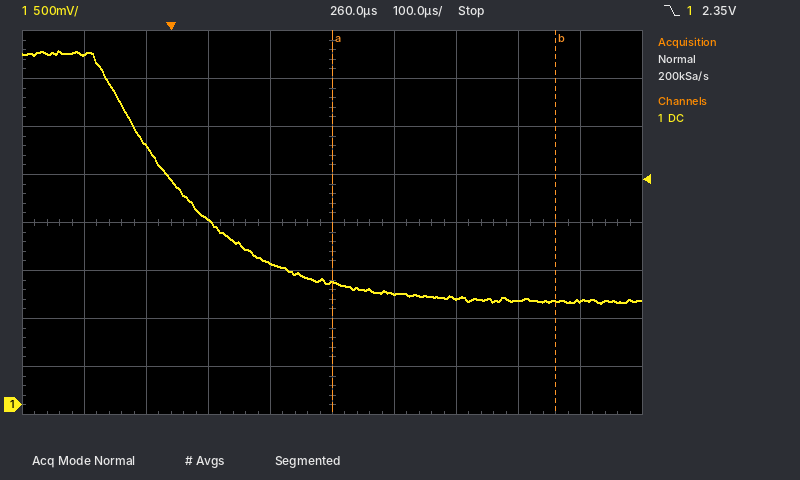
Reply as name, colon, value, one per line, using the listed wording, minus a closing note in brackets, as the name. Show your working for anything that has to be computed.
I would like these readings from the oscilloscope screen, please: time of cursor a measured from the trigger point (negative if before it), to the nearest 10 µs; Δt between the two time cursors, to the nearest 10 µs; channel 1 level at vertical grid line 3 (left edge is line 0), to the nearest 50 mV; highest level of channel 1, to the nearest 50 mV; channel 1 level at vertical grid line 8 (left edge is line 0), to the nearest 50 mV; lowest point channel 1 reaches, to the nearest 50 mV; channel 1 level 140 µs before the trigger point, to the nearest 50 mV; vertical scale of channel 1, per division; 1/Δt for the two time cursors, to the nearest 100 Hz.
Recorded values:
time of cursor a measured from the trigger point (negative if before it), to the nearest 10 µs: +260 µs
Δt between the two time cursors, to the nearest 10 µs: 360 µs
channel 1 level at vertical grid line 3 (left edge is line 0), to the nearest 50 mV: 1.95 V
highest level of channel 1, to the nearest 50 mV: 3.70 V
channel 1 level at vertical grid line 8 (left edge is line 0), to the nearest 50 mV: 1.10 V
lowest point channel 1 reaches, to the nearest 50 mV: 1.05 V
channel 1 level 140 µs before the trigger point, to the nearest 50 mV: 3.65 V
vertical scale of channel 1, per division: 500 mV
1/Δt for the two time cursors, to the nearest 100 Hz: 1 / 360 µs ≈ 2.8 kHz
